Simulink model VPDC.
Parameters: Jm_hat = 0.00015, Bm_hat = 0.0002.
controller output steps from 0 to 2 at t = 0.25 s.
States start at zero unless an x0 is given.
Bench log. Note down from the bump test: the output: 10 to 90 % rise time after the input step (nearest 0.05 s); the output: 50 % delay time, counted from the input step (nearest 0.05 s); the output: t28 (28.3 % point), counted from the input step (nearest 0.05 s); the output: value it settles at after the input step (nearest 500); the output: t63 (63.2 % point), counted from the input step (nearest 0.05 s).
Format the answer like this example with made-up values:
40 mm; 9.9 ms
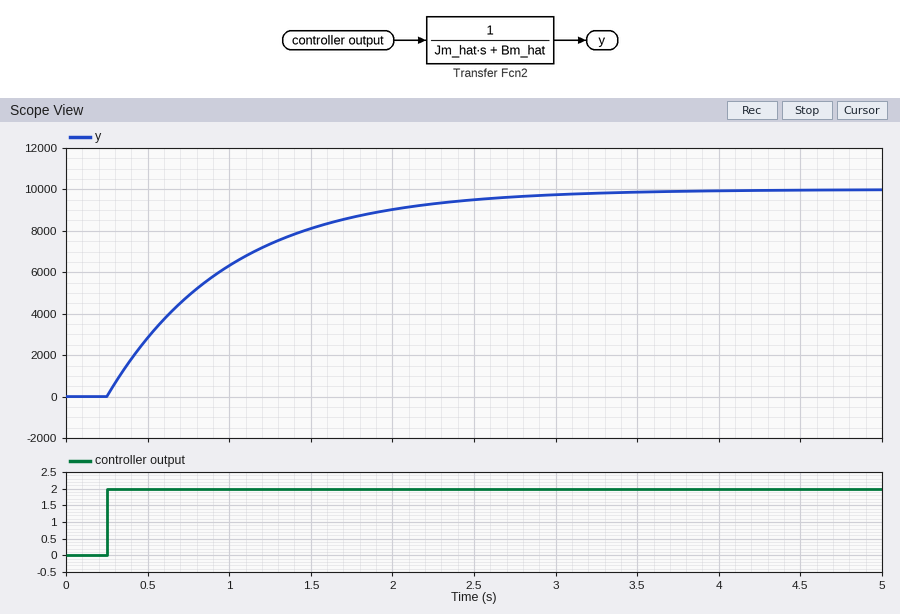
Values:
1.65 s; 0.50 s; 0.25 s; 10000; 0.75 s
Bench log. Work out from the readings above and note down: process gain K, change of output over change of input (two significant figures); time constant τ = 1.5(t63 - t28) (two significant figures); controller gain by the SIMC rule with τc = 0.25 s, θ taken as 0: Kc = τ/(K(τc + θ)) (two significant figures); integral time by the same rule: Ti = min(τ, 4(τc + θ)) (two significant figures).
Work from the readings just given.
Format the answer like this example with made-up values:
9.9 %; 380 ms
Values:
5000; 0.75 s; 0.00060; 0.75 s
